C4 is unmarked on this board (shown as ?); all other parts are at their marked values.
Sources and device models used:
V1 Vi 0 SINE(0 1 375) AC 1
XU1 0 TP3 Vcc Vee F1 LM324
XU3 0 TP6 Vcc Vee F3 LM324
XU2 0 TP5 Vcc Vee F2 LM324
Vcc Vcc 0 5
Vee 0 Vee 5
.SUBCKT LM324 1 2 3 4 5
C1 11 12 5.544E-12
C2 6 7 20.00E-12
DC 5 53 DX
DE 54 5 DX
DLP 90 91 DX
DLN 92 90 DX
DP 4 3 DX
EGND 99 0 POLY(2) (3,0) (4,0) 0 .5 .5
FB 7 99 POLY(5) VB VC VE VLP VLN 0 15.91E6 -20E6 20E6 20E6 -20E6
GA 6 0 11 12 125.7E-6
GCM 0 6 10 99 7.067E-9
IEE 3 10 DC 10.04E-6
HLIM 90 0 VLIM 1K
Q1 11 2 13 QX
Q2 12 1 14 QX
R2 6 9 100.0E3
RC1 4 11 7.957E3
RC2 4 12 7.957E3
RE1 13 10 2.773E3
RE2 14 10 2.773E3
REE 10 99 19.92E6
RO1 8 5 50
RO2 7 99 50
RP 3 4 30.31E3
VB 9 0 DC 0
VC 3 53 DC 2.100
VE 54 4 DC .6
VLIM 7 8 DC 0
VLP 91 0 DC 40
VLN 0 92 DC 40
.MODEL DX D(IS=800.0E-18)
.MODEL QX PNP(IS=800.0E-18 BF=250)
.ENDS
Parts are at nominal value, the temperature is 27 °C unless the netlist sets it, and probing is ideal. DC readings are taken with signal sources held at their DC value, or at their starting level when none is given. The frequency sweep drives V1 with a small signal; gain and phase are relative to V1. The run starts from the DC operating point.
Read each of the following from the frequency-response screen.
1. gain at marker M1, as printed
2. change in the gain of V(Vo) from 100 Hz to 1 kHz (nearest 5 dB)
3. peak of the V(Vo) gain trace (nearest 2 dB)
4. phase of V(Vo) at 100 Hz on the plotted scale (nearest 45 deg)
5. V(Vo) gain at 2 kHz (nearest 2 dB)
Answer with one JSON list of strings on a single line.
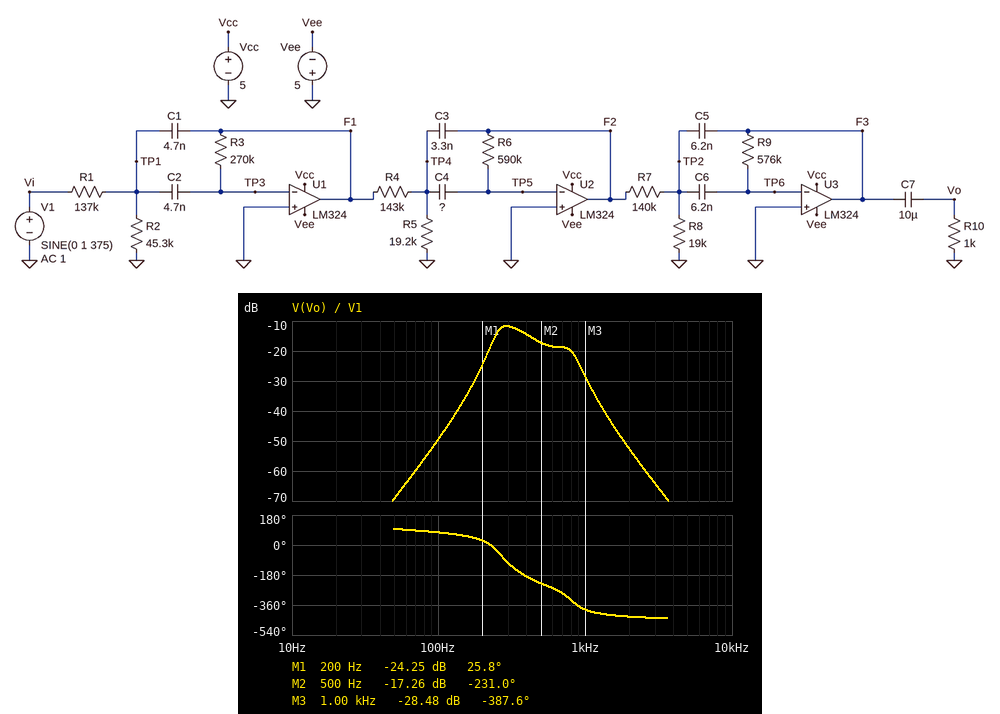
["-24.25 dB", "20 dB", "-12 dB", "90 deg", "-52 dB"]
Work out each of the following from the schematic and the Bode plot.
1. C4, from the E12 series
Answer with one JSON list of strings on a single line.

["1.2 nF"]
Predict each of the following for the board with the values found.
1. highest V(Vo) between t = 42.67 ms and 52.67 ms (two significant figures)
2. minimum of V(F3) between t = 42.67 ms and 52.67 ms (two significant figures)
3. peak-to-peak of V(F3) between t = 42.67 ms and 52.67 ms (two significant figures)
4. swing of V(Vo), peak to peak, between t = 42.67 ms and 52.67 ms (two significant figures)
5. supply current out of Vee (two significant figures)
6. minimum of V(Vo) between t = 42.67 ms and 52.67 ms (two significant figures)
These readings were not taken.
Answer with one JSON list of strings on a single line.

["210 mV", "-220 mV", "410 mV", "410 mV", "1.0 mA", "-210 mV"]
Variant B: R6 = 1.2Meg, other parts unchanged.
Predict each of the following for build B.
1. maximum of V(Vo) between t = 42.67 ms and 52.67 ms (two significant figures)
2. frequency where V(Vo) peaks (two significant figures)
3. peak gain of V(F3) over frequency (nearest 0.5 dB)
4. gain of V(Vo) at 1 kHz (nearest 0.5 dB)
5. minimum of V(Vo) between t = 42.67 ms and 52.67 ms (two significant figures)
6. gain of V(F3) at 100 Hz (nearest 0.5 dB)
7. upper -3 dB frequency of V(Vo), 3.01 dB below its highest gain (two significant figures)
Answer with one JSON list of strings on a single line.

["580 mV", "300 Hz", "-4.0 dB", "-32.0 dB", "-580 mV", "-43.0 dB", "590 Hz"]
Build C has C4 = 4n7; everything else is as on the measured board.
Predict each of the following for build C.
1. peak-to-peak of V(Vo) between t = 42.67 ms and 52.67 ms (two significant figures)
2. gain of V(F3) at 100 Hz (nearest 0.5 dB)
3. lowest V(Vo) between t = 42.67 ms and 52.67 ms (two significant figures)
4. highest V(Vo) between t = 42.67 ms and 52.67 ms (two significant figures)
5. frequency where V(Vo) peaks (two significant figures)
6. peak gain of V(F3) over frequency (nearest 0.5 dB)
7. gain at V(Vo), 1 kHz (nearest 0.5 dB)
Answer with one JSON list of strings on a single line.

["3.7 V", "-37.0 dB", "-1.9 V", "1.9 V", "360 Hz", "5.5 dB", "-33.5 dB"]
